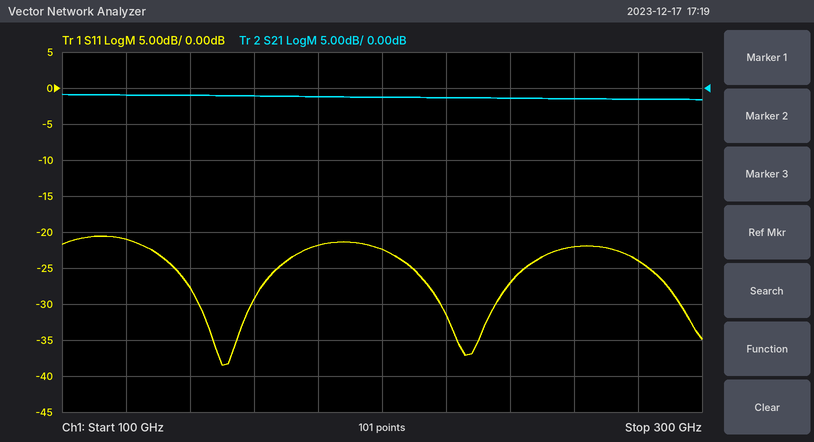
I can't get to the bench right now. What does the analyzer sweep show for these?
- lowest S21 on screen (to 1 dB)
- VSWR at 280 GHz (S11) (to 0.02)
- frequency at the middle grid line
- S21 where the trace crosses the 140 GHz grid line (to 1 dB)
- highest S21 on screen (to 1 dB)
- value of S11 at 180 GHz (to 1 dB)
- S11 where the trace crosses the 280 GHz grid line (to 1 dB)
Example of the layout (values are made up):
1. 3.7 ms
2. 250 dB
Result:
1. -2 dB
2. 1.14
3. 200 GHz
4. -1 dB
5. -1 dB
6. -22 dB
7. -24 dB
